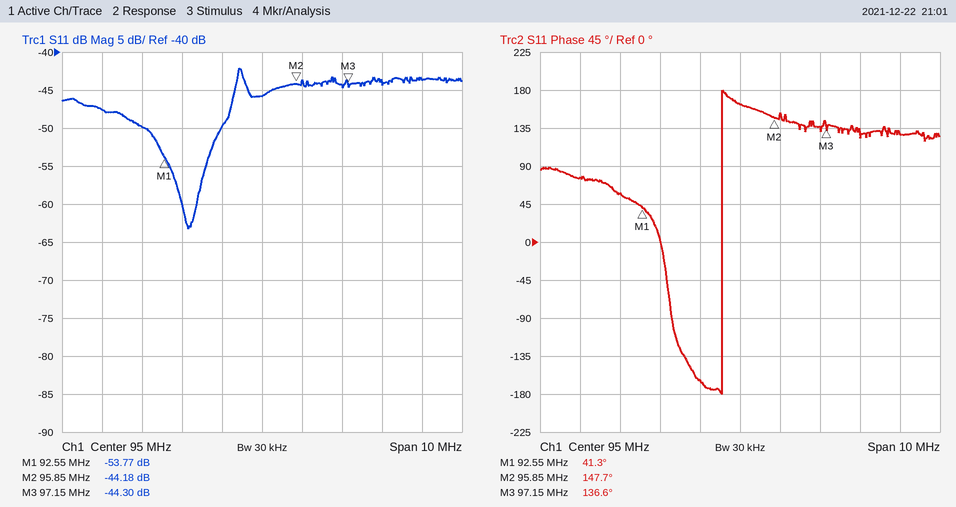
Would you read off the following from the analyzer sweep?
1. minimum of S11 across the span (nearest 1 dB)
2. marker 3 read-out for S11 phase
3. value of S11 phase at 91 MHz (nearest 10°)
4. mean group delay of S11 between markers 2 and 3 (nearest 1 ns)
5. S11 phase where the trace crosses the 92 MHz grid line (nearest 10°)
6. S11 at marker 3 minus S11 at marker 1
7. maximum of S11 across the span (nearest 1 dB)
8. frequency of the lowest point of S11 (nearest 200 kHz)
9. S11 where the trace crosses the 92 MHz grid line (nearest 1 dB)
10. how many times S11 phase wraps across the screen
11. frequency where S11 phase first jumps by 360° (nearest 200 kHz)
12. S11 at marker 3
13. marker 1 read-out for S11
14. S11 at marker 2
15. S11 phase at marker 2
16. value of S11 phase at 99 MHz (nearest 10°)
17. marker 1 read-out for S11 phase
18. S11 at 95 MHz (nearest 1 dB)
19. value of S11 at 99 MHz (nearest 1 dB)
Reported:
-63 dB
136.6°
80°
24 ns
60°
9.47 dB
-42 dB
93.2 MHz
-50 dB
1
94.6 MHz
-44.30 dB
-53.77 dB
-44.18 dB
147.7°
130°
41.3°
-46 dB
-44 dB
